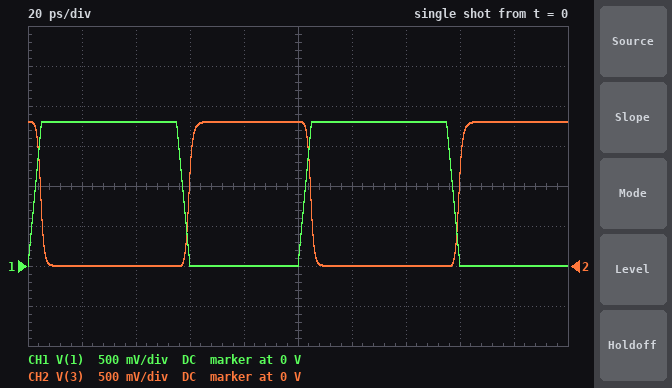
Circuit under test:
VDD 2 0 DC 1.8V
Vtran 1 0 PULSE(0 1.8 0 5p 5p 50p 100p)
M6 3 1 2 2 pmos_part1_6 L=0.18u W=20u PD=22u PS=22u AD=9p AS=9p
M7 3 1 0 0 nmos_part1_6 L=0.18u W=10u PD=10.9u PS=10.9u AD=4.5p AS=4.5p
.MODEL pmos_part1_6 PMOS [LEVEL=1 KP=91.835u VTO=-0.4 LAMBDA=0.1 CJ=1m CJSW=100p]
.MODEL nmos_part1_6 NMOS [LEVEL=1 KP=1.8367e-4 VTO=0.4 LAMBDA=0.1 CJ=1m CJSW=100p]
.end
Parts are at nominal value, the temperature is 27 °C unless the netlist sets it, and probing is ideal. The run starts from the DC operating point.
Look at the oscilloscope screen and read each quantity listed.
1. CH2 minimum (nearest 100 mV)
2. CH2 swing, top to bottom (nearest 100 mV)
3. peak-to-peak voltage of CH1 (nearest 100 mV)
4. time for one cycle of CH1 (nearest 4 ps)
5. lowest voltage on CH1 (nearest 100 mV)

0 V
1.8 V
1.8 V
100 ps
0 V
